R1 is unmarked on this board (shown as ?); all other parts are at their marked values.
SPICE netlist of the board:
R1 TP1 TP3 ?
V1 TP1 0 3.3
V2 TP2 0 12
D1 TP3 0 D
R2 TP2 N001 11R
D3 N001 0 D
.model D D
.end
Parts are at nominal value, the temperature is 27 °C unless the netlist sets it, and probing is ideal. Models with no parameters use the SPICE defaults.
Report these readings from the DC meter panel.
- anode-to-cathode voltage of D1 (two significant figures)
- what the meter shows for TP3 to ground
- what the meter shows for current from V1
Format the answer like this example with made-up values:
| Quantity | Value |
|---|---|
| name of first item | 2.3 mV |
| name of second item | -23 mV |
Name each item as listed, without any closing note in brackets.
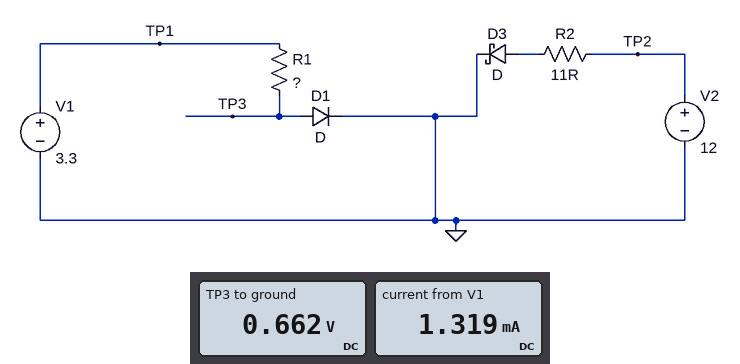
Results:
| Quantity | Value |
|---|---|
| anode-to-cathode voltage of D1 | 660 mV |
| what the meter shows for TP3 to ground | 0.662 V |
| what the meter shows for current from V1 | 1.319 mA |
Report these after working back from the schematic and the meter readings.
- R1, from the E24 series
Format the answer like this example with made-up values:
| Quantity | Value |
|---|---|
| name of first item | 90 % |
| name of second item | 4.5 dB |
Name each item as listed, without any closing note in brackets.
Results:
| Quantity | Value |
|---|---|
| R1, from the E24 series | 2 kΩ |
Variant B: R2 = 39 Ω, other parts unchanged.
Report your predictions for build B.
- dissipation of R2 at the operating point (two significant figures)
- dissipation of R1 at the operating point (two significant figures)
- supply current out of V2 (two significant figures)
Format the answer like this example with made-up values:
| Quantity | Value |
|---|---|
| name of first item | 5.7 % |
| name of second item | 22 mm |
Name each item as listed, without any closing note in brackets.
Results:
| Quantity | Value |
|---|---|
| dissipation of R2 at the operating point | 3.2 W |
| dissipation of R1 at the operating point | 3.5 mW |
| supply current out of V2 | 290 mA |
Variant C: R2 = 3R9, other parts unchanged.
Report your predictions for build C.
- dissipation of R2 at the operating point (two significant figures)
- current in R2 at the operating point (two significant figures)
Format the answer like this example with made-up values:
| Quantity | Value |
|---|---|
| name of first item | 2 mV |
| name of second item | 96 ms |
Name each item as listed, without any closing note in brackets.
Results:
| Quantity | Value |
|---|---|
| dissipation of R2 at the operating point | 32 W |
| current in R2 at the operating point | 2.9 A |
